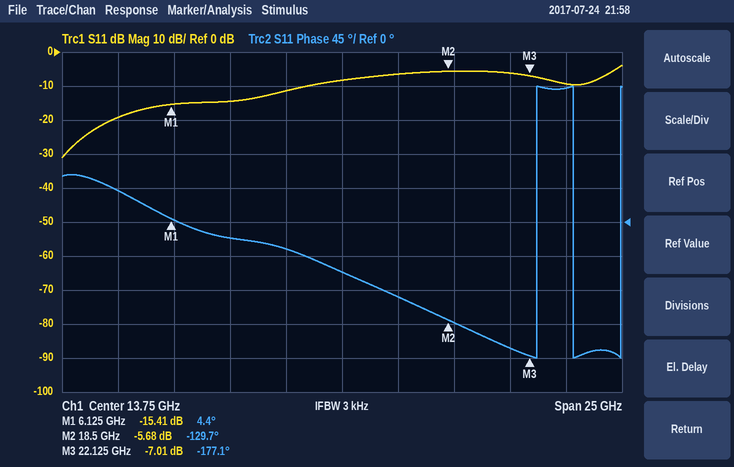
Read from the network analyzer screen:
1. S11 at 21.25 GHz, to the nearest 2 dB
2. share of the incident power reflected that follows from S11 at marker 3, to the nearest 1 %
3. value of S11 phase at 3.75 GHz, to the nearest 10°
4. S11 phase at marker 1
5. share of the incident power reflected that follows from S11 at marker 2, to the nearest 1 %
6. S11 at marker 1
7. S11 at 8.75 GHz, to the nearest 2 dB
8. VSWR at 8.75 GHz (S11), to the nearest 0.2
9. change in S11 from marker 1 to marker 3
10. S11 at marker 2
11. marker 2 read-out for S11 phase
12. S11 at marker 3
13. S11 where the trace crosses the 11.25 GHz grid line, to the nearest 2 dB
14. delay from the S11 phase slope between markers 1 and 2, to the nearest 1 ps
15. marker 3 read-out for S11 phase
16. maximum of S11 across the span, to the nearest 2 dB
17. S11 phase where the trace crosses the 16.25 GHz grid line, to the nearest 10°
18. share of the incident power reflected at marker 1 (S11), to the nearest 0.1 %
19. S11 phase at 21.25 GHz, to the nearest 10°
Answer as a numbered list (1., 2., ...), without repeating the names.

1. -6 dB
2. 20 %
3. 40°
4. 4.4°
5. 27 %
6. -15.41 dB
7. -14 dB
8. 1.4
9. 8.40 dB
10. -5.68 dB
11. -129.7°
12. -7.01 dB
13. -12 dB
14. 30 ps
15. -177.1°
16. -4 dB
17. -100°
18. 2.9 %
19. -170°
